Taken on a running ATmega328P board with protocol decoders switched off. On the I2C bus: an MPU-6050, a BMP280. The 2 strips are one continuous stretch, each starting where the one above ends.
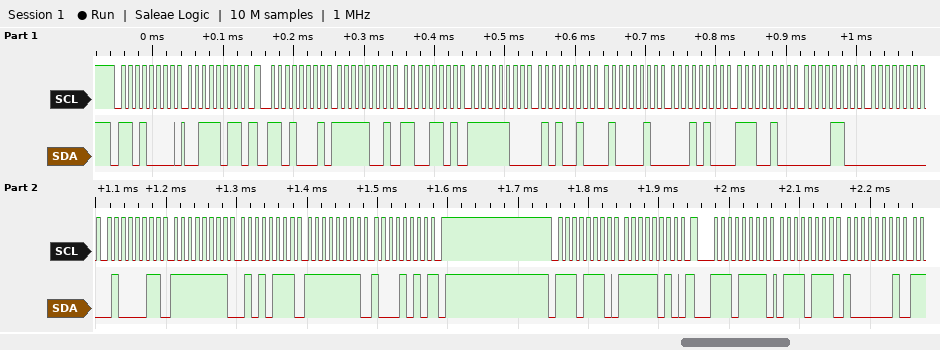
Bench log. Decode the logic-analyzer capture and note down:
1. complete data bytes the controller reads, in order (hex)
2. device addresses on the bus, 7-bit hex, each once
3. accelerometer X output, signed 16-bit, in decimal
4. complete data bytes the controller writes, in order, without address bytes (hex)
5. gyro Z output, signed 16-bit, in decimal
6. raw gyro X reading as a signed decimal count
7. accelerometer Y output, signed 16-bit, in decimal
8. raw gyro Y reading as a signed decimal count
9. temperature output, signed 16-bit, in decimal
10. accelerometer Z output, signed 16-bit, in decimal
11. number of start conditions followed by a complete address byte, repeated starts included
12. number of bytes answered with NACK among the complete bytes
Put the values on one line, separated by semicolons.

F9 CD FC 52 42 14 E4 0C 00 43 FF 57 FF 8A 77 81; 0x68 0x77; -1587; 3B FA; -118; 67; -942; -169; -7156; 16916; 4; 1
